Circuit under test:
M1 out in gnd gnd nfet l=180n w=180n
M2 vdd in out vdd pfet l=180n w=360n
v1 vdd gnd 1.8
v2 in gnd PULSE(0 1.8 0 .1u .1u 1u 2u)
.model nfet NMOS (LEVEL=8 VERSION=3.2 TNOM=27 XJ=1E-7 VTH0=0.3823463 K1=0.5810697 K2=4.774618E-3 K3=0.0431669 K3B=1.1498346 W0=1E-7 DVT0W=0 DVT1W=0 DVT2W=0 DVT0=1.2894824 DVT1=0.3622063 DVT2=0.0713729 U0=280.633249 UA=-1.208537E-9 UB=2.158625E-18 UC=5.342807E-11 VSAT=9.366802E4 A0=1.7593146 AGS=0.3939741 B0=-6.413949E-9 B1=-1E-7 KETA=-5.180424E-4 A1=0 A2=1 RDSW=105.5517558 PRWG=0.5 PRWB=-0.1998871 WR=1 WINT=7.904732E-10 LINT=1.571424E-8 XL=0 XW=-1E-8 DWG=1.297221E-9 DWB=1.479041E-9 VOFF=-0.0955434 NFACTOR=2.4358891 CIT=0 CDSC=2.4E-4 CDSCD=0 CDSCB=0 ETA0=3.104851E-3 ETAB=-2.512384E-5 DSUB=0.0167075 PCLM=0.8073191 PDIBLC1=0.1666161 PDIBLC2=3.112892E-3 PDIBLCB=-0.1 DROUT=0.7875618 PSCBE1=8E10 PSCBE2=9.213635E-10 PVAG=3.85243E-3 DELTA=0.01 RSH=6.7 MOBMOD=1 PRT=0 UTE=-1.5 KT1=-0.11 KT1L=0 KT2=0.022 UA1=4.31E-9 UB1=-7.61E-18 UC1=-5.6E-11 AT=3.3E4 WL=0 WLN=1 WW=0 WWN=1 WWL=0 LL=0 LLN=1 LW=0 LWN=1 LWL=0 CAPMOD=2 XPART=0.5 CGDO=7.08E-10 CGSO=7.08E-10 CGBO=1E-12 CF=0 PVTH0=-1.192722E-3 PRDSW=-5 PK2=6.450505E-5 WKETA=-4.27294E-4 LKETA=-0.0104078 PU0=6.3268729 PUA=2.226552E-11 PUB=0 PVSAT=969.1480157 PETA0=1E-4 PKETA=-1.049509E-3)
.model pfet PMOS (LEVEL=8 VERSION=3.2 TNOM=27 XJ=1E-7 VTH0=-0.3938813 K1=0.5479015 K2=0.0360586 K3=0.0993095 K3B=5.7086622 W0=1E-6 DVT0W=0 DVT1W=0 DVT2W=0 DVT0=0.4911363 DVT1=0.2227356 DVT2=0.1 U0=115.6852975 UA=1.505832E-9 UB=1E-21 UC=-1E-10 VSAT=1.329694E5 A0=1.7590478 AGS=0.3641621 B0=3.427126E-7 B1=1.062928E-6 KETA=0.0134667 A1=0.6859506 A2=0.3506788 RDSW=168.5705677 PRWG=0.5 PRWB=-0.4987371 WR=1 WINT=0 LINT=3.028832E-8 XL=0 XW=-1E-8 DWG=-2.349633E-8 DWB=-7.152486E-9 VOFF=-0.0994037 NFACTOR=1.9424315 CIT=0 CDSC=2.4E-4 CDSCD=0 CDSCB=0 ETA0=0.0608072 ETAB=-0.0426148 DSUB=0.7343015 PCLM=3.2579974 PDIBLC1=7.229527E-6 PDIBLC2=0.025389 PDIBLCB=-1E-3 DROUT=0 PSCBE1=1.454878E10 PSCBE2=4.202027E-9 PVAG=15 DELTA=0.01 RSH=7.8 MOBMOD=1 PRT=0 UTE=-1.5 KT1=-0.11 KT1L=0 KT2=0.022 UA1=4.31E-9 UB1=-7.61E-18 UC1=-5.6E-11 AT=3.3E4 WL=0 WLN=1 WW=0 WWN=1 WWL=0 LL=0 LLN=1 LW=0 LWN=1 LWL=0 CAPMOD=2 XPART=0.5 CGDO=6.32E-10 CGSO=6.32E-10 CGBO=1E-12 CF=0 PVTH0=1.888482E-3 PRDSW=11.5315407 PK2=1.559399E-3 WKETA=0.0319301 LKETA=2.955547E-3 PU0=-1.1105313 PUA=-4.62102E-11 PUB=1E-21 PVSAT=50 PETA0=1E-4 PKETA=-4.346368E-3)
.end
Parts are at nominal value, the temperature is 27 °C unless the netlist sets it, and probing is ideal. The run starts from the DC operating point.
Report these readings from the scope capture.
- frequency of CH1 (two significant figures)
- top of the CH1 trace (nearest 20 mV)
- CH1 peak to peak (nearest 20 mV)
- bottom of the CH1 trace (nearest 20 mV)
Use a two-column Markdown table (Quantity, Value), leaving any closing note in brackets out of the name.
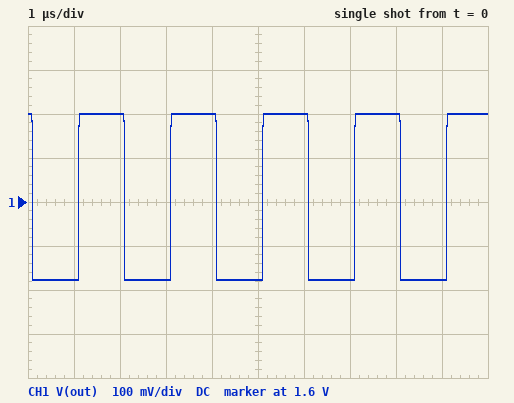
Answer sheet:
| Quantity | Value |
|---|---|
| frequency of CH1 | 500 kHz |
| top of the CH1 trace | 1.80 V |
| CH1 peak to peak | 380 mV |
| bottom of the CH1 trace | 1.42 V |
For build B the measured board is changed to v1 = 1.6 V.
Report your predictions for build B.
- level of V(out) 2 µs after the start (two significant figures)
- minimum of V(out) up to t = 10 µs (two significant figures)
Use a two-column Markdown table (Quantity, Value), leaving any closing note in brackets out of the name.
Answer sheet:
| Quantity | Value |
|---|---|
| level of V(out) 2 µs after the start | 1.6 V |
| minimum of V(out) up to t = 10 µs | 18 mV |
